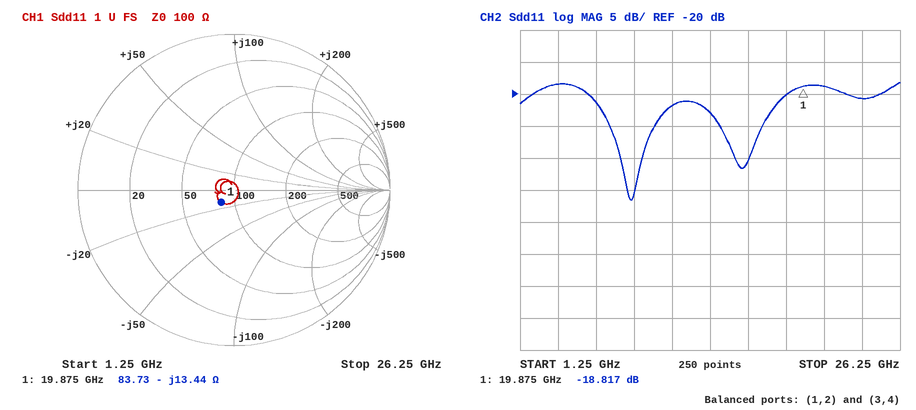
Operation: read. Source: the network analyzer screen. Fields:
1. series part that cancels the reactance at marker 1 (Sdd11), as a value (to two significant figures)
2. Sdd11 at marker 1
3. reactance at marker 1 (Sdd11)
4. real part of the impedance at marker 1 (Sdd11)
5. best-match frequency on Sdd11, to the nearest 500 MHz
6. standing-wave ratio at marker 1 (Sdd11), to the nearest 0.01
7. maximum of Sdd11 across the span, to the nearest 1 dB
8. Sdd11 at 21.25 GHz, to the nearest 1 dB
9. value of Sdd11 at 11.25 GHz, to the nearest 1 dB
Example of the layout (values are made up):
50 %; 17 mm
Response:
110 pH; -18.817 dB; -13.44 Ω; 83.73 Ω; 8.5 GHz; 1.26; -18 dB; -19 dB; -22 dB
